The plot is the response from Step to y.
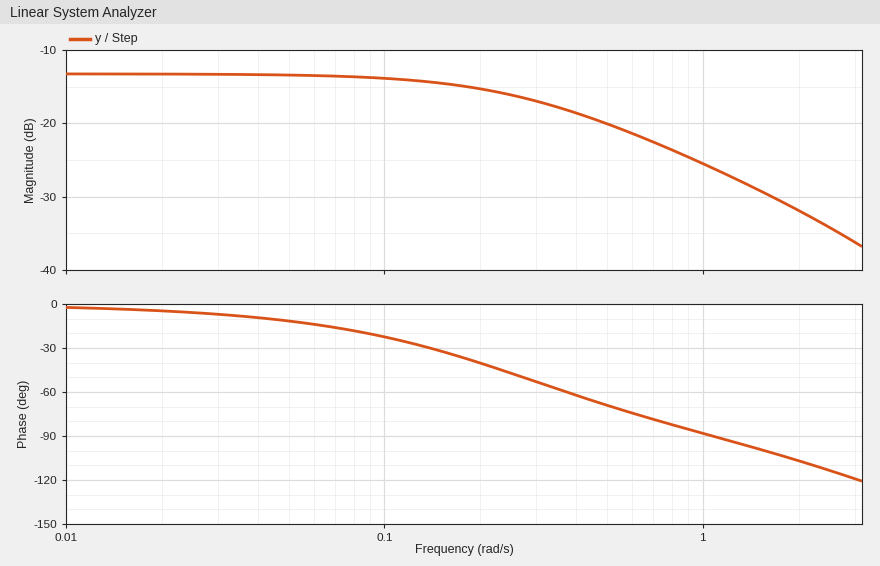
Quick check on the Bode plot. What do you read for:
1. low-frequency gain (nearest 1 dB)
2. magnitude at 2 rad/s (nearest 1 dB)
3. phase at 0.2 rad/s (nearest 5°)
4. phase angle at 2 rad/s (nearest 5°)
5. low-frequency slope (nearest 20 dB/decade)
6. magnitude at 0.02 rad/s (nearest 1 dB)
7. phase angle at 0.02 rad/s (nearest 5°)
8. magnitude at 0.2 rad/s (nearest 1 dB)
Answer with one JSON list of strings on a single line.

["-13 dB", "-32 dB", "-40°", "-105°", "0 dB/decade", "-13 dB", "-5°", "-15 dB"]
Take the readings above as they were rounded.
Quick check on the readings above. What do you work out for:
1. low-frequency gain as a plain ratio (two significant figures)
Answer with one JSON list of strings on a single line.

["0.22"]
